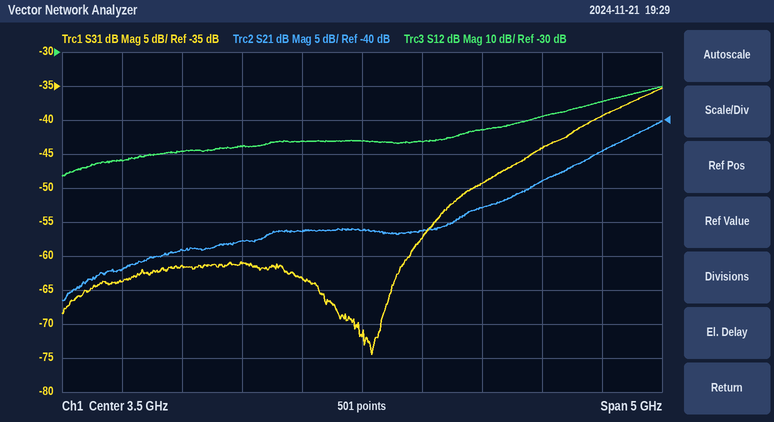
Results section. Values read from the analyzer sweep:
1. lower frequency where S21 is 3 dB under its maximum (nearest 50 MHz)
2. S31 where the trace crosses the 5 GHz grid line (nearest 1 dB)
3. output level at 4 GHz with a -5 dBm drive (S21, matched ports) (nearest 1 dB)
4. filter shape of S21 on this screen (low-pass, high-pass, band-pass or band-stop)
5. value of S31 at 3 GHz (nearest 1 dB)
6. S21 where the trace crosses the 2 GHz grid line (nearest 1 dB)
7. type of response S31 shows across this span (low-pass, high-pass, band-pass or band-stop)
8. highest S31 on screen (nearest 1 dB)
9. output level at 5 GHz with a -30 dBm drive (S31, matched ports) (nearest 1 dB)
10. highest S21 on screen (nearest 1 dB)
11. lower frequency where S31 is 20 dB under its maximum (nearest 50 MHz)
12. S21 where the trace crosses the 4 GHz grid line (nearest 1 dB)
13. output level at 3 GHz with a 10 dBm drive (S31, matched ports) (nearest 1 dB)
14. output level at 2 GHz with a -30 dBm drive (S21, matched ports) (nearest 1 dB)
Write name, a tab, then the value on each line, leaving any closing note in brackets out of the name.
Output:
lower frequency where S21 is 3 dB under its maximum	5.65 GHz
S31 where the trace crosses the 5 GHz grid line	-44 dB
output level at 4 GHz with a -5 dBm drive (S21, matched ports)	-61 dBm
filter shape of S21 on this screen	high-pass
value of S31 at 3 GHz	-63 dB
S21 where the trace crosses the 2 GHz grid line	-59 dB
type of response S31 shows across this span	high-pass
highest S31 on screen	-35 dB
output level at 5 GHz with a -30 dBm drive (S31, matched ports)	-74 dBm
highest S21 on screen	-40 dB
lower frequency where S31 is 20 dB under its maximum	4.10 GHz
S21 where the trace crosses the 4 GHz grid line	-56 dB
output level at 3 GHz with a 10 dBm drive (S31, matched ports)	-53 dBm
output level at 2 GHz with a -30 dBm drive (S21, matched ports)	-89 dBm
